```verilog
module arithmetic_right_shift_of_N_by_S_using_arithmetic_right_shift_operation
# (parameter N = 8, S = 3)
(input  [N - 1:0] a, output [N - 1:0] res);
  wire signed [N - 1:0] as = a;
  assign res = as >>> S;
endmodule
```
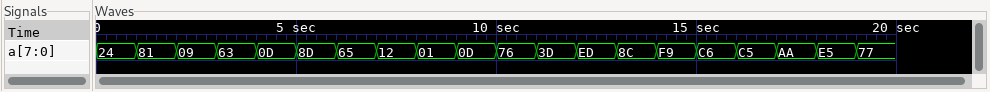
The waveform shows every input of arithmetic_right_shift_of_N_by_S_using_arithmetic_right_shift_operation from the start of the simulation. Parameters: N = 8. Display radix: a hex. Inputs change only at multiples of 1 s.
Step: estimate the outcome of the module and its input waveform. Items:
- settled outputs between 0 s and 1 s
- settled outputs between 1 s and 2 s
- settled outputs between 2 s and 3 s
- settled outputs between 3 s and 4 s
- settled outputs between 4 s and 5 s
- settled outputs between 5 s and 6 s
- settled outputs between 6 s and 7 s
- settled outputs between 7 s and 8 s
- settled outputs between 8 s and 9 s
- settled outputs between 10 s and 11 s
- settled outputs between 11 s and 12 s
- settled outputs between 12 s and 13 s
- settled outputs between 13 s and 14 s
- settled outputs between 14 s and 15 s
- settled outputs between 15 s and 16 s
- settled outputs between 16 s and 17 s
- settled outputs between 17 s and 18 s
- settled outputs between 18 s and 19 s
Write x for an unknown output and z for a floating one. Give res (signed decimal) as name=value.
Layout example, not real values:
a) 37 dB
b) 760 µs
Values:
a) res=4
b) res=-16
c) res=1
d) res=12
e) res=1
f) res=-15
g) res=12
h) res=2
i) res=0
j) res=14
k) res=7
l) res=-3
m) res=-15
n) res=-1
o) res=-8
p) res=-8
q) res=-11
r) res=-4
